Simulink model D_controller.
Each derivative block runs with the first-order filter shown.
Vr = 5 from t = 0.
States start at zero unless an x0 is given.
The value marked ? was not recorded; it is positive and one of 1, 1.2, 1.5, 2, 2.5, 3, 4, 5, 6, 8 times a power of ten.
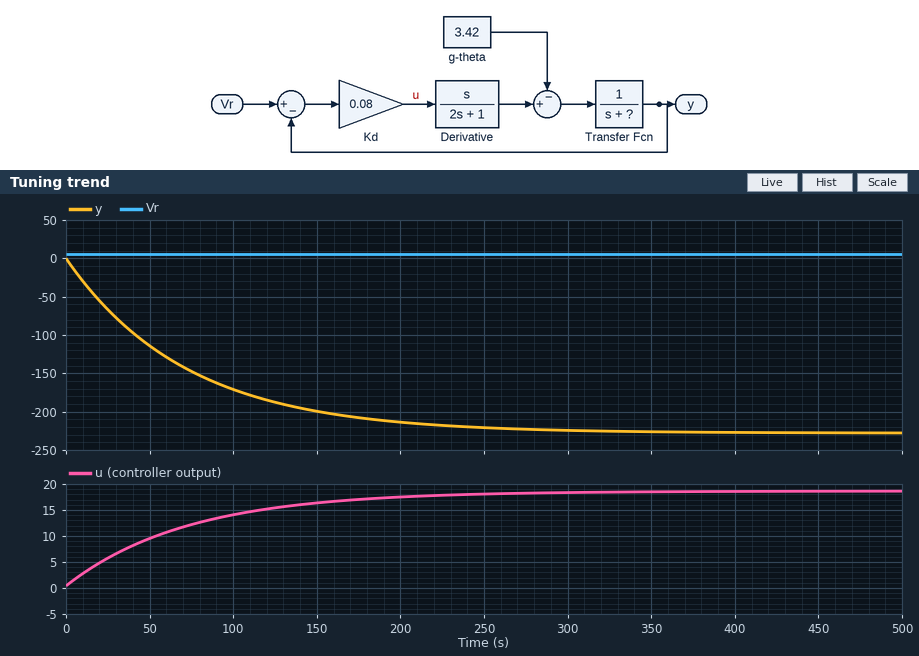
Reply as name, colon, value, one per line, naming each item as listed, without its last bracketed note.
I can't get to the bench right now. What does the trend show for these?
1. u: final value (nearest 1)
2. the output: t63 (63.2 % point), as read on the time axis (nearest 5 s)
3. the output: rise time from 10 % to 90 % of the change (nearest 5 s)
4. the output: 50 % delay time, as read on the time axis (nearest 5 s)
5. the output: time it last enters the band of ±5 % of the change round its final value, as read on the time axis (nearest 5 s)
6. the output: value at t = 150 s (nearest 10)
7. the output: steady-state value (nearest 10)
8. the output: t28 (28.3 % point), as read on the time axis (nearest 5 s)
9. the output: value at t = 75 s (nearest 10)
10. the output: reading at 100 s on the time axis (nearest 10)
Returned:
u: final value: 19
the output: t63 (63.2 % point), as read on the time axis: 70 s
the output: rise time from 10 % to 90 % of the change: 160 s
the output: 50 % delay time, as read on the time axis: 50 s
the output: time it last enters the band of ±5 % of the change round its final value, as read on the time axis: 215 s
the output: value at t = 150 s: -200
the output: steady-state value: -230
the output: t28 (28.3 % point), as read on the time axis: 25 s
the output: value at t = 75 s: -150
the output: reading at 100 s on the time axis: -170
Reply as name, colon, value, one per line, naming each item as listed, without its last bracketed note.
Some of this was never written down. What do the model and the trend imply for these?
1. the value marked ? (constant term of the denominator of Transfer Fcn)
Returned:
the value marked ?: 0.015
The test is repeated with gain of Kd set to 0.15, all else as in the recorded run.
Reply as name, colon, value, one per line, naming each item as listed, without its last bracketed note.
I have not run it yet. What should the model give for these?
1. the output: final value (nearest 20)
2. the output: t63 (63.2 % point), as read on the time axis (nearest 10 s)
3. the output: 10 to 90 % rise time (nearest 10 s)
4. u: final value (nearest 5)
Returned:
the output: final value: -220
the output: t63 (63.2 % point), as read on the time axis: 80 s
the output: 10 to 90 % rise time: 170 s
u: final value: 35
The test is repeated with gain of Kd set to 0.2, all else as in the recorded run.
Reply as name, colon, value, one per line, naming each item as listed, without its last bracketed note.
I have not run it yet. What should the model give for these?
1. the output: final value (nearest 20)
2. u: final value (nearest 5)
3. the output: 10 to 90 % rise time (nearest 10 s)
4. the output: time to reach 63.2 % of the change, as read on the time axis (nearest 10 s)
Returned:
the output: final value: -220
u: final value: 45
the output: 10 to 90 % rise time: 180 s
the output: time to reach 63.2 % of the change, as read on the time axis: 80 s
